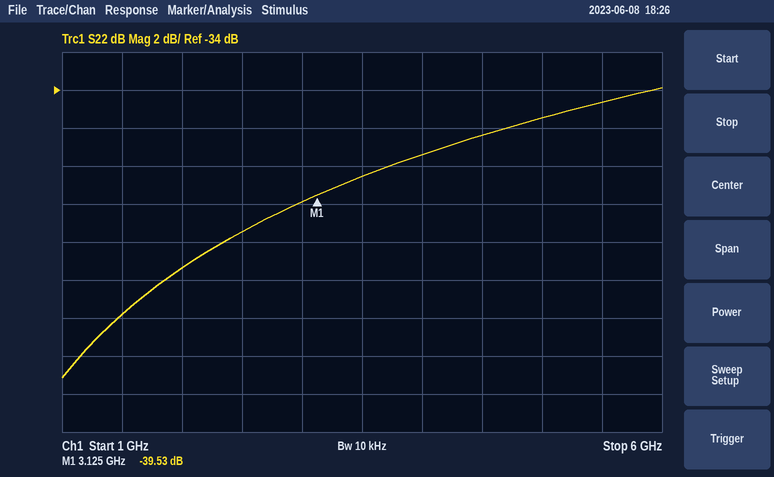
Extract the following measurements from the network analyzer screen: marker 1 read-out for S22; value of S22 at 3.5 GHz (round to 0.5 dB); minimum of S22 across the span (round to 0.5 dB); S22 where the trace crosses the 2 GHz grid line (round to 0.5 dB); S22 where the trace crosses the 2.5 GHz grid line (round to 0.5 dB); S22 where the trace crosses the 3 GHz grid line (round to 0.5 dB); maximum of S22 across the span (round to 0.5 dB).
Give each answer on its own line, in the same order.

-39.53 dB
-38.5 dB
-49.0 dB
-43.5 dB
-41.5 dB
-40.0 dB
-34.0 dB
